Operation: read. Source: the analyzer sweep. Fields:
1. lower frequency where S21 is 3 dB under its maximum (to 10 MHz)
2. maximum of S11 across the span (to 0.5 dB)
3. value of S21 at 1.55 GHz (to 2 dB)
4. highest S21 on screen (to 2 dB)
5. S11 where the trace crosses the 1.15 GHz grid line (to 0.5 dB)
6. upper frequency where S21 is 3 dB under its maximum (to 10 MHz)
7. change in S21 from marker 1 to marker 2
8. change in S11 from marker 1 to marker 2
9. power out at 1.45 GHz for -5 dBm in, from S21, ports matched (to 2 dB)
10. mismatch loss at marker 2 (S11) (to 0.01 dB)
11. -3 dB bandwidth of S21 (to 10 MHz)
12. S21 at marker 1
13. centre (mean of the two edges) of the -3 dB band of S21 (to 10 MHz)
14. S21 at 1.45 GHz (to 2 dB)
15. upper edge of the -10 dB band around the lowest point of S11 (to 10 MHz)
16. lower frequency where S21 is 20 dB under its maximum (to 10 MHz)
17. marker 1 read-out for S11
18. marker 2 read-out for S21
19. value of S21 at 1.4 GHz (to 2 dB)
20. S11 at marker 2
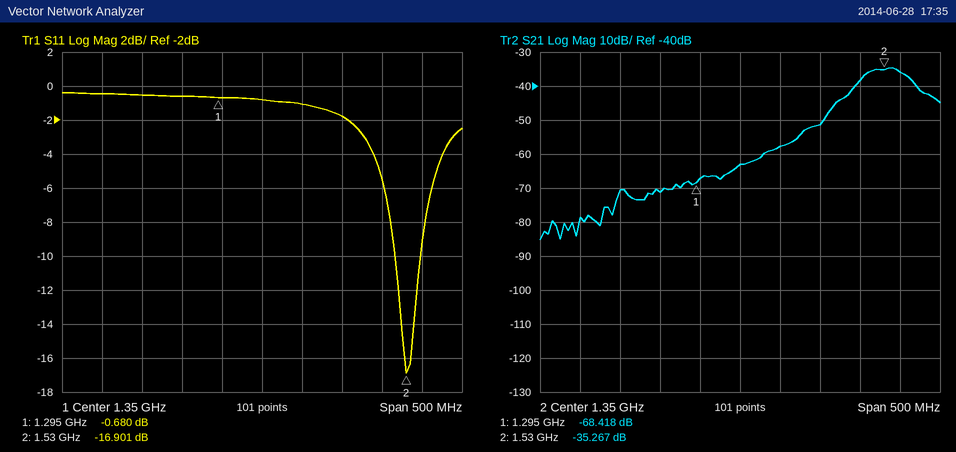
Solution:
1.50 GHz
-0.5 dB
-36 dB
-34 dB
-0.5 dB
1.56 GHz
33.151 dB
-16.221 dB
-56 dBm
0.09 dB
60 MHz
-68.418 dB
1.53 GHz
-52 dB
1.55 GHz
1.42 GHz
-0.680 dB
-35.267 dB
-58 dB
-16.901 dB
